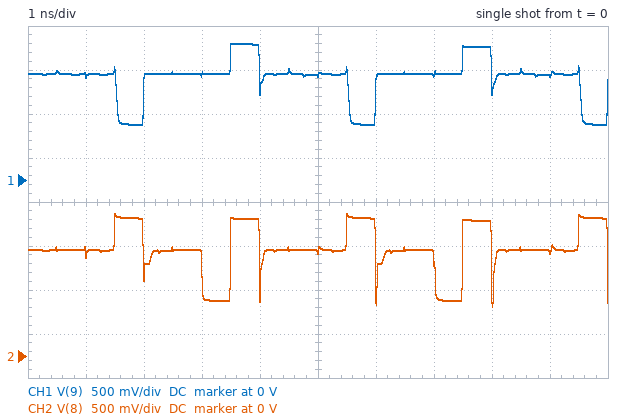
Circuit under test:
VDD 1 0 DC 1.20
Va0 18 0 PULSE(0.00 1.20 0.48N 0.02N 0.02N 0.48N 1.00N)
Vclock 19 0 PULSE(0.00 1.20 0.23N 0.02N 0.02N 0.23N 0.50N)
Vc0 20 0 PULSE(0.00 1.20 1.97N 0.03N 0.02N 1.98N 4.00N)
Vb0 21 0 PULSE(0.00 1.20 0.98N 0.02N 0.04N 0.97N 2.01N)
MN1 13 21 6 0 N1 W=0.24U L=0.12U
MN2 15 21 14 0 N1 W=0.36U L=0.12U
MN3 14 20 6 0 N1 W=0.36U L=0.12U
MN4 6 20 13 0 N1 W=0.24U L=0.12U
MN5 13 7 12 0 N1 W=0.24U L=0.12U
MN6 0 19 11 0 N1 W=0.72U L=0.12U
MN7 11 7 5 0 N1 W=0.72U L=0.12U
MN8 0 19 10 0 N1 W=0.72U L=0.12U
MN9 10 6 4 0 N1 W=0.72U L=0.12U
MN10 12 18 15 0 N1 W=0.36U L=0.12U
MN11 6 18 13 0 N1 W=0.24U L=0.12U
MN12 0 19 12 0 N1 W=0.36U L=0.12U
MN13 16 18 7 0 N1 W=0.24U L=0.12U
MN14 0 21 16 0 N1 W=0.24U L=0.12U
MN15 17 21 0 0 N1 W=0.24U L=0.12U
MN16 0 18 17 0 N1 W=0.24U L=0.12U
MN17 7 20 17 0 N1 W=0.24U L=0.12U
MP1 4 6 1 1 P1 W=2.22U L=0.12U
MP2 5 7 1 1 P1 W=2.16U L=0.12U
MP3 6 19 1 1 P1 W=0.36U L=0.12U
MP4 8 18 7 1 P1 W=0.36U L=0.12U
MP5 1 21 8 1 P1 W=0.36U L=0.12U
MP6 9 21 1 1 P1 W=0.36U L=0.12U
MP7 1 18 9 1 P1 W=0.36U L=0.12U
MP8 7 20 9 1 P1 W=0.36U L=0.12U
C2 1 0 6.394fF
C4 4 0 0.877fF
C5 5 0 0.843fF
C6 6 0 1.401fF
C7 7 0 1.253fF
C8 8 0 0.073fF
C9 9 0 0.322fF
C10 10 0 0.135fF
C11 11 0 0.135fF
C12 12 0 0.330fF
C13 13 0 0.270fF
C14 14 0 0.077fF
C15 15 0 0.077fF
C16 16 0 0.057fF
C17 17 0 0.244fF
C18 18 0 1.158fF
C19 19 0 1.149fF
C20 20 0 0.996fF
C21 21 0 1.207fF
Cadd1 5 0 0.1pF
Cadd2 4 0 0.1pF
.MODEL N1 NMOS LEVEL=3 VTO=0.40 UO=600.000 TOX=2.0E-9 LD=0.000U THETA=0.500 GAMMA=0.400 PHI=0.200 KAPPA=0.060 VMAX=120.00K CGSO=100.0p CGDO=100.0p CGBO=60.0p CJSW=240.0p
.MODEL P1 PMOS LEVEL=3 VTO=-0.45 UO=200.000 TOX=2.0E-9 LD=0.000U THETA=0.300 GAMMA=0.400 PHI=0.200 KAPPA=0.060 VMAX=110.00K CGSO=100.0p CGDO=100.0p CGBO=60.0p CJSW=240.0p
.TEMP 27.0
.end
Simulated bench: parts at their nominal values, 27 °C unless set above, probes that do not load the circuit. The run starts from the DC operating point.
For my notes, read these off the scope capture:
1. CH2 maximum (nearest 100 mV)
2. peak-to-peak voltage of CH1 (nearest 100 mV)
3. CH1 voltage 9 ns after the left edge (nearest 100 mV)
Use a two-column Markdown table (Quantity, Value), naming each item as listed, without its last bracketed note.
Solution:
| Quantity | Value |
|---|---|
| CH2 maximum | 1.6 V |
| peak-to-peak voltage of CH1 | 900 mV |
| CH1 voltage 9 ns after the left edge | 1.2 V |
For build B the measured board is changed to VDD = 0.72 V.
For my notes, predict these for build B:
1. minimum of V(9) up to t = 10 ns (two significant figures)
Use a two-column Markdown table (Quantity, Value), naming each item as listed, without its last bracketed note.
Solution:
| Quantity | Value |
|---|---|
| minimum of V(9) up to t = 10 ns | 530 mV |
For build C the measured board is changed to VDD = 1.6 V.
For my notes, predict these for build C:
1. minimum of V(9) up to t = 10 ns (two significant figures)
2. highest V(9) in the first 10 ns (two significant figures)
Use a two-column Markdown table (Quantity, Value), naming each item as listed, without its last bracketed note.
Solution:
| Quantity | Value |
|---|---|
| minimum of V(9) up to t = 10 ns | 700 mV |
| highest V(9) in the first 10 ns | 1.7 V |
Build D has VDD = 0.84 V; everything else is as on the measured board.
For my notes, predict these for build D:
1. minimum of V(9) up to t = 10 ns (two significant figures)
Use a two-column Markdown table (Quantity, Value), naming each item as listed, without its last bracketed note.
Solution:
| Quantity | Value |
|---|---|
| minimum of V(9) up to t = 10 ns | 550 mV |
